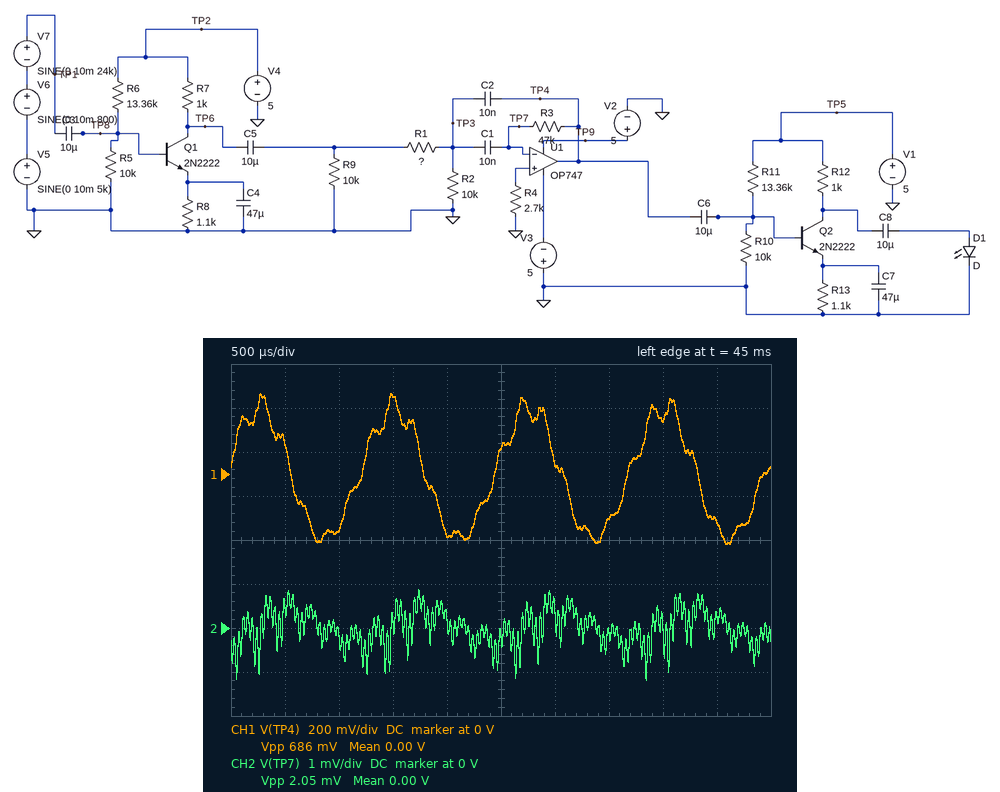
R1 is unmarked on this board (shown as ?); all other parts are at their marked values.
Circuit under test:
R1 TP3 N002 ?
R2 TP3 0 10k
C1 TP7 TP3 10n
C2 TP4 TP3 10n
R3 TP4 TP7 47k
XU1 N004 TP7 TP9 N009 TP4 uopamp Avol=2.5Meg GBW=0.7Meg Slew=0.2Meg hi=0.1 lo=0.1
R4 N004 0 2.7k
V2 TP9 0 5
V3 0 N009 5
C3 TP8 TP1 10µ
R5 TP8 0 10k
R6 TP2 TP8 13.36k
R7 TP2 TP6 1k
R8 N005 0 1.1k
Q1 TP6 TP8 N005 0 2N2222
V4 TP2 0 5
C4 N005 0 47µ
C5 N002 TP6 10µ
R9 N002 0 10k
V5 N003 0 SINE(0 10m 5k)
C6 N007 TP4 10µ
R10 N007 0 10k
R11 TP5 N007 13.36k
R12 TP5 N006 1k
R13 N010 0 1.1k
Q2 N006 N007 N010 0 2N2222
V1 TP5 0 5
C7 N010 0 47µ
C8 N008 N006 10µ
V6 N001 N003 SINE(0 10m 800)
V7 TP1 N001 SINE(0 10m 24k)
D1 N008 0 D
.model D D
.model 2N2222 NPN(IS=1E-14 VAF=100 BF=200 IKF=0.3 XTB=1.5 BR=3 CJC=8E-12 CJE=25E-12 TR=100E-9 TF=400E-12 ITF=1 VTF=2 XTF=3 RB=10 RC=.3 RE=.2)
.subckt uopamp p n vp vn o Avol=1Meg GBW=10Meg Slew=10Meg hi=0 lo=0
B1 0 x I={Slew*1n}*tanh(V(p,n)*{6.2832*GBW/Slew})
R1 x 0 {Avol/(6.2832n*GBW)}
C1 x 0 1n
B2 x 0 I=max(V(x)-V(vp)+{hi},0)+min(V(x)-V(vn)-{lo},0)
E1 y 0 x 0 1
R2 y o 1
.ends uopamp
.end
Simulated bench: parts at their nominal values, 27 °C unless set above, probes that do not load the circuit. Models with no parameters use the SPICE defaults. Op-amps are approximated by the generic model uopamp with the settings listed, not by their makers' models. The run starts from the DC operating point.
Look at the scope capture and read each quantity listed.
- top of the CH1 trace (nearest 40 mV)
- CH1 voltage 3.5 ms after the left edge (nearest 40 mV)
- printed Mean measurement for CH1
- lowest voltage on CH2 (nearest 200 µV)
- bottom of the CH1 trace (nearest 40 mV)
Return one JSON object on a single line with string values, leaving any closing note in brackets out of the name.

{"top of the CH1 trace": "360 mV", "CH1 voltage 3.5 ms after the left edge": "-200 mV", "printed Mean measurement for CH1": "0.00 V", "lowest voltage on CH2": "-1.2 mV", "bottom of the CH1 trace": "-320 mV"}
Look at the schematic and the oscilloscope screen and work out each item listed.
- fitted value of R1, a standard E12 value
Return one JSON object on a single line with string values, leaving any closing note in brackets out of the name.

{"fitted value of R1, a standard E12 value": "33 kΩ"}
